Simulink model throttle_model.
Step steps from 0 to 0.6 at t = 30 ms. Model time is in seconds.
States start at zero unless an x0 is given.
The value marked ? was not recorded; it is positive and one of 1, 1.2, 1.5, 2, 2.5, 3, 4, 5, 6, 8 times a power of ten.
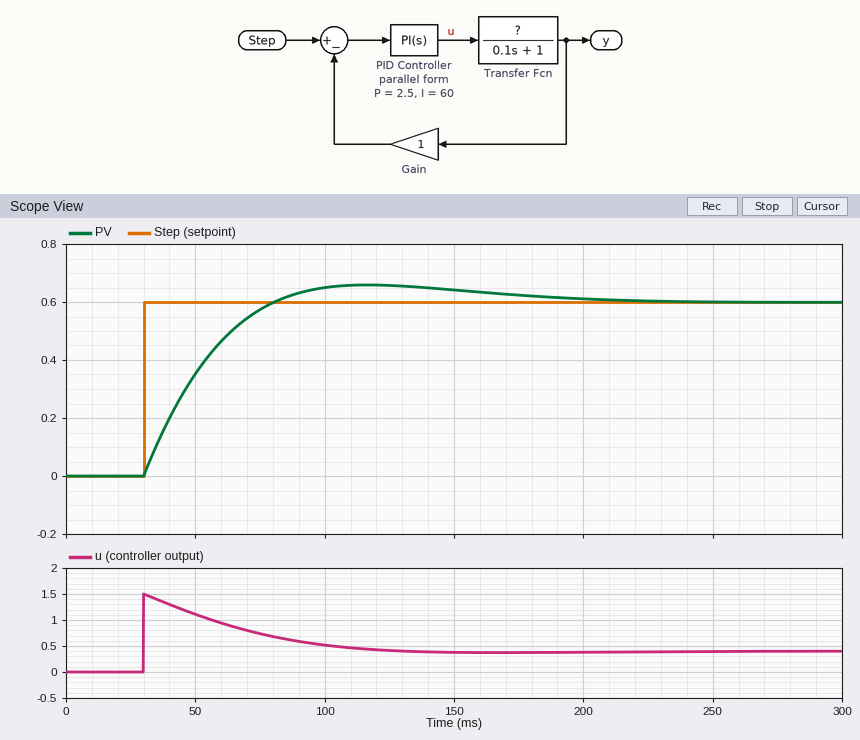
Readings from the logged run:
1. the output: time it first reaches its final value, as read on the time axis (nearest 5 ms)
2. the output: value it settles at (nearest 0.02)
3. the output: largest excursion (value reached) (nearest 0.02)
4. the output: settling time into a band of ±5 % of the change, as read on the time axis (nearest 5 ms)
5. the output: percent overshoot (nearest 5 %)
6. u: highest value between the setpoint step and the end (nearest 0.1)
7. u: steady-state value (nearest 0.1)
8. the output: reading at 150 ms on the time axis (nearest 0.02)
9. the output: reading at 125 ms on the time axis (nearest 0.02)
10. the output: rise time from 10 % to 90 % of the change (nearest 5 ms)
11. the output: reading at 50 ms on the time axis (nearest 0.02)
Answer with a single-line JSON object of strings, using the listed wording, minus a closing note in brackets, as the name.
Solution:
{"the output: time it first reaches its final value, as read on the time axis": "80 ms", "the output: value it settles at": "0.60", "the output: largest excursion (value reached)": "0.66", "the output: settling time into a band of ±5 % of the change, as read on the time axis": "165 ms", "the output: percent overshoot": "10 %", "u: highest value between the setpoint step and the end": "1.5", "u: steady-state value": "0.4", "the output: reading at 150 ms on the time axis": "0.64", "the output: reading at 125 ms on the time axis": "0.66", "the output: rise time from 10 % to 90 % of the change": "35 ms", "the output: reading at 50 ms on the time axis": "0.36"}
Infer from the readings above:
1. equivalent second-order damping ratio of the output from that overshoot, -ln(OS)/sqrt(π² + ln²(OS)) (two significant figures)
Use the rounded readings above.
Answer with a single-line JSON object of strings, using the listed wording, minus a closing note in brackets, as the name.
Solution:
{"equivalent second-order damping ratio of the output from that overshoot, -ln(OS)/sqrt(π² + ln²(OS))": "0.59"}
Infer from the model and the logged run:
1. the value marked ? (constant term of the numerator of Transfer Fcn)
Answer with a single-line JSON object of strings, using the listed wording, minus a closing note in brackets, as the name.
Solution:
{"the value marked ?": "1.5"}
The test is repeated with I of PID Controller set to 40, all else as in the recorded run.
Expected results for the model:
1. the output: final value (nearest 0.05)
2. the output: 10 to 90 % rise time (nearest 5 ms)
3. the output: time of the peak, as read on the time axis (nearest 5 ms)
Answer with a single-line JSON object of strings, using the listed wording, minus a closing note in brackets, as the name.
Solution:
{"the output: final value": "0.60", "the output: 10 to 90 % rise time": "45 ms", "the output: time of the peak, as read on the time axis": "140 ms"}
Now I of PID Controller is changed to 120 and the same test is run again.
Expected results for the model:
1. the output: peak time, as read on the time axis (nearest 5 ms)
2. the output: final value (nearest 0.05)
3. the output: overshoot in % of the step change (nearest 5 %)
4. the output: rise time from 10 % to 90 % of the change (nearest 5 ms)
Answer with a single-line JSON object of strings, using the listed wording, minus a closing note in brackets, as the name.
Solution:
{"the output: peak time, as read on the time axis": "90 ms", "the output: final value": "0.60", "the output: overshoot in % of the step change": "20 %", "the output: rise time from 10 % to 90 % of the change": "25 ms"}
